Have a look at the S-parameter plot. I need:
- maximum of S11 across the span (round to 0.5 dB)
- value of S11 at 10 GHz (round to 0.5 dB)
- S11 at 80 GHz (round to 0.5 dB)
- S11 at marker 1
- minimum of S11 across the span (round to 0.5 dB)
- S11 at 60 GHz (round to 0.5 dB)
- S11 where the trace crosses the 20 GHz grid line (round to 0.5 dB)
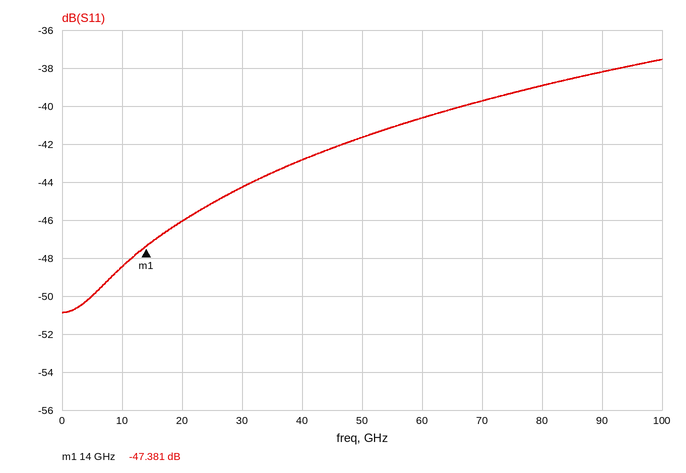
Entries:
-37.5 dB
-48.5 dB
-39.0 dB
-47.381 dB
-51.0 dB
-40.5 dB
-46.0 dB
